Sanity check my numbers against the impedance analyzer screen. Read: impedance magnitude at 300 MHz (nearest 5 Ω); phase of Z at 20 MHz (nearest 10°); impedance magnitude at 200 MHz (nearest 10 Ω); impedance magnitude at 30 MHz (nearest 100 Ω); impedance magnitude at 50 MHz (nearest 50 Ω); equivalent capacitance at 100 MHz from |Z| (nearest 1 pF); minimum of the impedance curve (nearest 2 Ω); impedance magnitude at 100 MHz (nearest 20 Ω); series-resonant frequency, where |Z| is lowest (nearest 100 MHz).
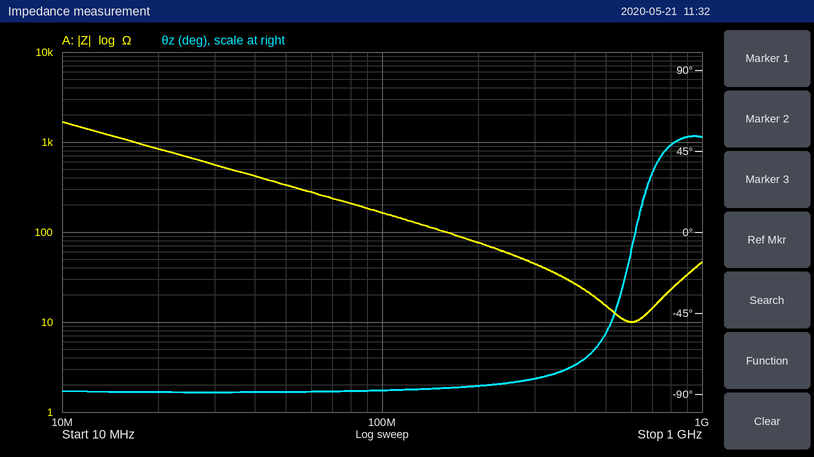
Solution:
45 Ω
-90°
80 Ω
600 Ω
350 Ω
10 pF
10 Ω
160 Ω
600 MHz
